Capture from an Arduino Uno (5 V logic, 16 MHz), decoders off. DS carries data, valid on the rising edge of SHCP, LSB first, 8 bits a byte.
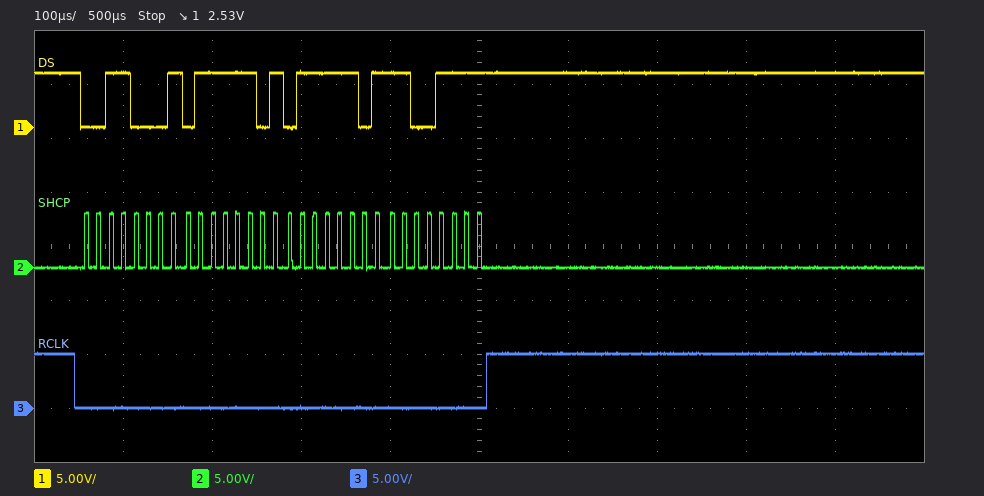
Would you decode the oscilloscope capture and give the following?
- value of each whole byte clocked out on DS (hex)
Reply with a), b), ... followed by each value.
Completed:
a) 8C BE BE F3
